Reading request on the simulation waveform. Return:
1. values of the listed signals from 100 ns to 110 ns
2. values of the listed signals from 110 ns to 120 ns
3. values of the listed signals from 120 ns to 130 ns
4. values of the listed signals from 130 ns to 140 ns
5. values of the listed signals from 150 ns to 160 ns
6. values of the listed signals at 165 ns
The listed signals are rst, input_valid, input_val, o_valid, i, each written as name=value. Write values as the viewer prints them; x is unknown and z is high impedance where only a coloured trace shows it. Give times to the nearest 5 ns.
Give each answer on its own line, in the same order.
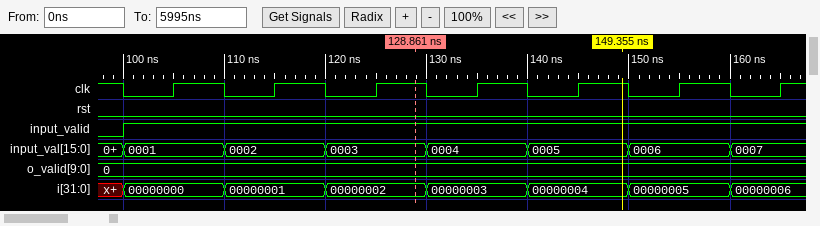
rst=0, input_valid=1, input_val=0001, o_valid=0, i=00000000
rst=0, input_valid=1, input_val=0002, o_valid=0, i=00000001
rst=0, input_valid=1, input_val=0003, o_valid=0, i=00000002
rst=0, input_valid=1, input_val=0004, o_valid=0, i=00000003
rst=0, input_valid=1, input_val=0006, o_valid=0, i=00000005
rst=0, input_valid=1, input_val=0007, o_valid=0, i=00000006
